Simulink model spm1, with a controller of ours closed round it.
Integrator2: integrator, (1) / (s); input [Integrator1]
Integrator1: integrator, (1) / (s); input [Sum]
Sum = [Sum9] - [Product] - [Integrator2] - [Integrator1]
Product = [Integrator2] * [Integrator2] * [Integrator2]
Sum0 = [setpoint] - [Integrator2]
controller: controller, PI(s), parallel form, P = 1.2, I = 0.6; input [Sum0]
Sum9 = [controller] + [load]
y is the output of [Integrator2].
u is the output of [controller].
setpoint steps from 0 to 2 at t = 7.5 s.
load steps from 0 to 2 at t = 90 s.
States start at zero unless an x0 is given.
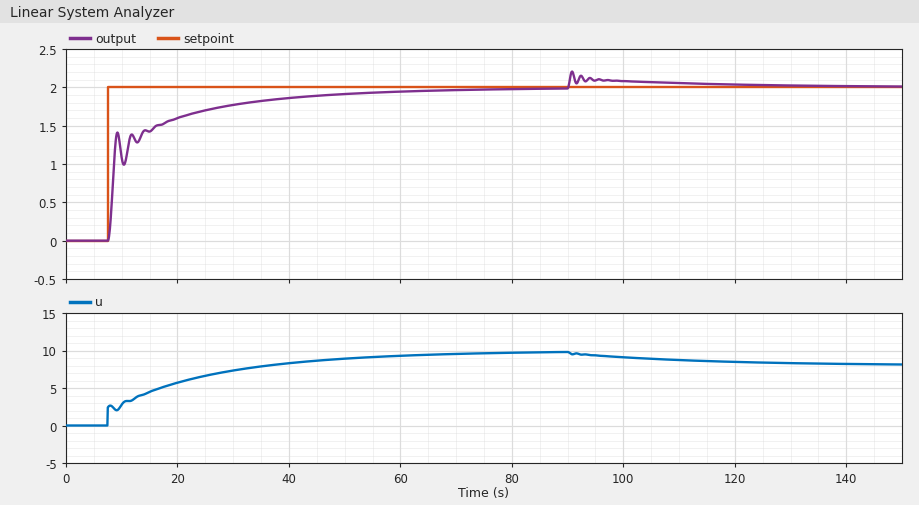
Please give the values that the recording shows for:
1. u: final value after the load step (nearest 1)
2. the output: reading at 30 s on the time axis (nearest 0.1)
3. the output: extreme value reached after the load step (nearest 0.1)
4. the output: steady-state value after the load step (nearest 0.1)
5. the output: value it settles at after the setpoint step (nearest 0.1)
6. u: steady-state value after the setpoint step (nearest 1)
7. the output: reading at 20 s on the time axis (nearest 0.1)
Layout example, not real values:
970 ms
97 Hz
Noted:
8
1.8
2.2
2.0
2.0
10
1.6
